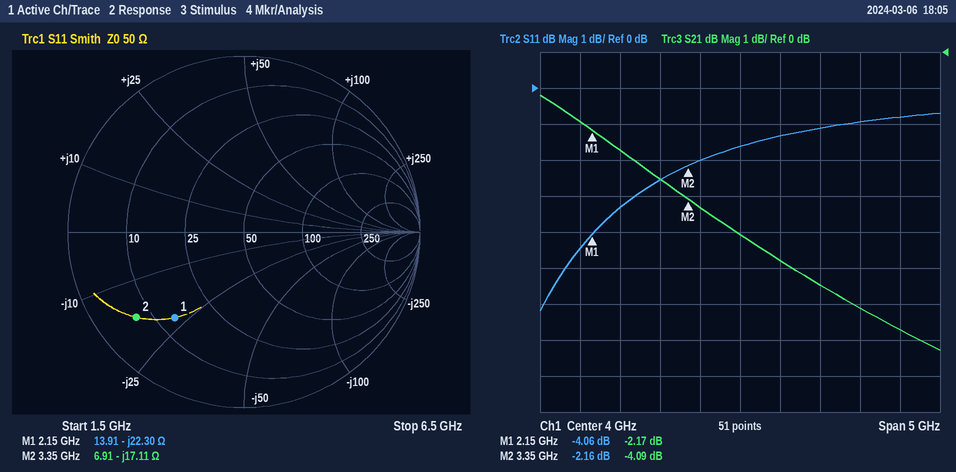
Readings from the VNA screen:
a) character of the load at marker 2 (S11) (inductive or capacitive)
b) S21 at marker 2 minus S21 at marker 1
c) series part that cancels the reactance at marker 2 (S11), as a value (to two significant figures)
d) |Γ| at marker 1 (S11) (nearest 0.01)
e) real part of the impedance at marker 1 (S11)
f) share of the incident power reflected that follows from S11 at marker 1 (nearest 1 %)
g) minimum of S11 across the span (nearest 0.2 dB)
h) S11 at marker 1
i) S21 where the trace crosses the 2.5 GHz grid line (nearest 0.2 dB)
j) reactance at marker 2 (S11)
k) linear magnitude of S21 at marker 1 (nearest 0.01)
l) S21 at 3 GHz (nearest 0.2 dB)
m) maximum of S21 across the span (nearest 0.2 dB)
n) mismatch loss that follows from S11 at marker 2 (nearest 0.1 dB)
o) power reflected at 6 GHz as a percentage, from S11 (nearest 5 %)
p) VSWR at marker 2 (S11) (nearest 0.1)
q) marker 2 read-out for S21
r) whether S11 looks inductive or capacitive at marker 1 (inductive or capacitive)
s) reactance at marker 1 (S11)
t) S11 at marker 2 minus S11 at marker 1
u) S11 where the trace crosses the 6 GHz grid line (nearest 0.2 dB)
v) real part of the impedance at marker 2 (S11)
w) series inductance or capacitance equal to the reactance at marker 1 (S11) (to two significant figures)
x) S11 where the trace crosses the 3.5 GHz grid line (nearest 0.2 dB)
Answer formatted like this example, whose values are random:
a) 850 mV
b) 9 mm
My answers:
a) capacitive
b) -1.92 dB
c) 810 pH
d) 0.63
e) 13.91 Ω
f) 39 %
g) -6.2 dB
h) -4.06 dB
i) -2.8 dB
j) -17.11 Ω
k) 0.78
l) -3.6 dB
m) -1.2 dB
n) 4.1 dB
o) 85 %
p) 8.1
q) -4.09 dB
r) capacitive
s) -22.30 Ω
t) 1.90 dB
u) -0.8 dB
v) 6.91 Ω
w) 3.3 pF
x) -2.0 dB
